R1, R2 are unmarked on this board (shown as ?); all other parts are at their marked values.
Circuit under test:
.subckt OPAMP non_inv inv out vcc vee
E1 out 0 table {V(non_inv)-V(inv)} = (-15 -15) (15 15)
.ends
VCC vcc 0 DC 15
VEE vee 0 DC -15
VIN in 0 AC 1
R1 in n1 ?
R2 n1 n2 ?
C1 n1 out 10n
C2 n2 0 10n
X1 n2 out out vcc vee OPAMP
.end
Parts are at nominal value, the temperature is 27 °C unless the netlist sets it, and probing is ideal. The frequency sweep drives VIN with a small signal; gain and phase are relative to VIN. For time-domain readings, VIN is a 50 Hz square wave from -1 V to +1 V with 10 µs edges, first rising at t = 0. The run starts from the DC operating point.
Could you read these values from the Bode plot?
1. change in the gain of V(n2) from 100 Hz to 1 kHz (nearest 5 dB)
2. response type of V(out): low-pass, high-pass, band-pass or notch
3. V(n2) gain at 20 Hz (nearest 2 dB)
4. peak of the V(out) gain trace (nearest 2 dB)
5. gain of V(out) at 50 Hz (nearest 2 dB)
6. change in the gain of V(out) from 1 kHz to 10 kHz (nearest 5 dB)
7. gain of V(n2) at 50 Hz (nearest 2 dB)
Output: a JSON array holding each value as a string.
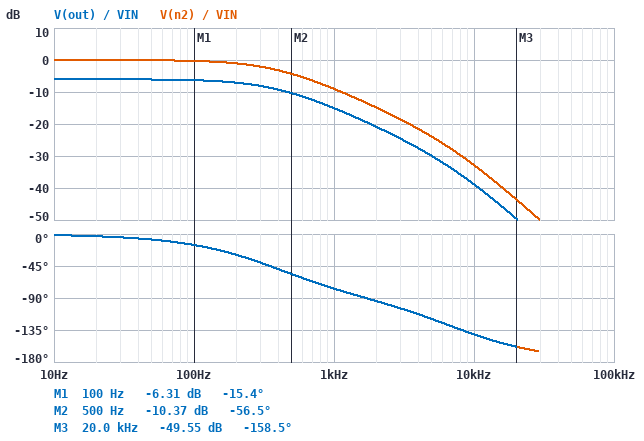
["-10 dB", "low-pass", "0 dB", "-6 dB", "-6 dB", "-25 dB", "0 dB"]
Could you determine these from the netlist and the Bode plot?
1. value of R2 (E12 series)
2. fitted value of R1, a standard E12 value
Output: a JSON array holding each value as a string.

["3.3 kΩ", "27 kΩ"]
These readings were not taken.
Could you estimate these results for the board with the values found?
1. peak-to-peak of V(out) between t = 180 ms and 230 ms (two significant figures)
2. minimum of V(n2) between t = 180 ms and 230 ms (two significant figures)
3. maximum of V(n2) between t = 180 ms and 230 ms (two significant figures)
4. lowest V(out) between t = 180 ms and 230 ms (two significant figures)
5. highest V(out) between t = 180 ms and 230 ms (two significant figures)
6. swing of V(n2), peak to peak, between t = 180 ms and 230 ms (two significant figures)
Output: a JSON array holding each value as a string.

["1.0 V", "-1.0 V", "1.0 V", "-500 mV", "500 mV", "2.0 V"]
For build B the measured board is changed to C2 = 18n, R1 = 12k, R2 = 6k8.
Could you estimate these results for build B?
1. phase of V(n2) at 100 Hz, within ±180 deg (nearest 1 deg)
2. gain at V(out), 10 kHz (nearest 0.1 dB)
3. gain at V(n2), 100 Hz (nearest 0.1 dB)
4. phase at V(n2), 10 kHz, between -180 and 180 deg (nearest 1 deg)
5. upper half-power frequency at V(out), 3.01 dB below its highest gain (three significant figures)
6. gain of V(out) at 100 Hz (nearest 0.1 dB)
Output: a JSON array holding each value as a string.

["-14 deg", "-41.9 dB", "-0.2 dB", "-156 deg", "440 Hz", "-6.2 dB"]
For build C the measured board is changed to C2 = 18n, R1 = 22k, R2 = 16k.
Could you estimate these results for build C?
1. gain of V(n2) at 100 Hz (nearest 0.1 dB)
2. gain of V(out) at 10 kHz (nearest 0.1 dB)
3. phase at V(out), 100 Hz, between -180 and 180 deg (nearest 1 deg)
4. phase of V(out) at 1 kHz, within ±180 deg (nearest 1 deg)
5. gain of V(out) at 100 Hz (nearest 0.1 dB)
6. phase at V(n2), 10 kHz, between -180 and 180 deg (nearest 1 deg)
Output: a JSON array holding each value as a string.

["-0.8 dB", "-54.1 dB", "-27 deg", "-107 deg", "-6.8 dB", "-169 deg"]
